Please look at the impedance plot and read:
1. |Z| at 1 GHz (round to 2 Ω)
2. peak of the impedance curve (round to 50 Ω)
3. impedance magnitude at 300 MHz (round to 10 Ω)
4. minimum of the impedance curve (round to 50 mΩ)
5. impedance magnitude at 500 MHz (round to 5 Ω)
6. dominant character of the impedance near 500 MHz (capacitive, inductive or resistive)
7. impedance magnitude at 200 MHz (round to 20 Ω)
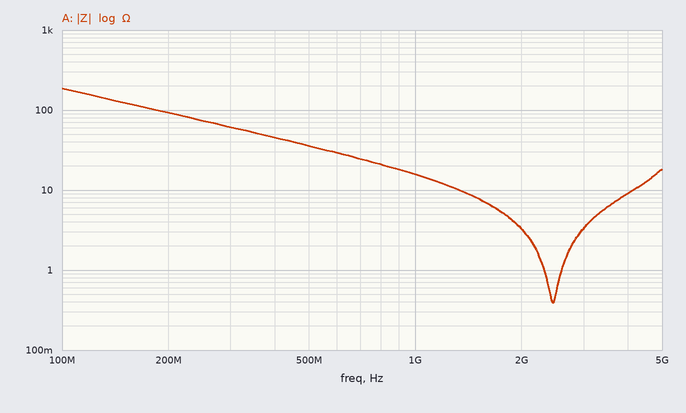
16 Ω
200 Ω
60 Ω
400 mΩ
35 Ω
capacitive
100 Ω
